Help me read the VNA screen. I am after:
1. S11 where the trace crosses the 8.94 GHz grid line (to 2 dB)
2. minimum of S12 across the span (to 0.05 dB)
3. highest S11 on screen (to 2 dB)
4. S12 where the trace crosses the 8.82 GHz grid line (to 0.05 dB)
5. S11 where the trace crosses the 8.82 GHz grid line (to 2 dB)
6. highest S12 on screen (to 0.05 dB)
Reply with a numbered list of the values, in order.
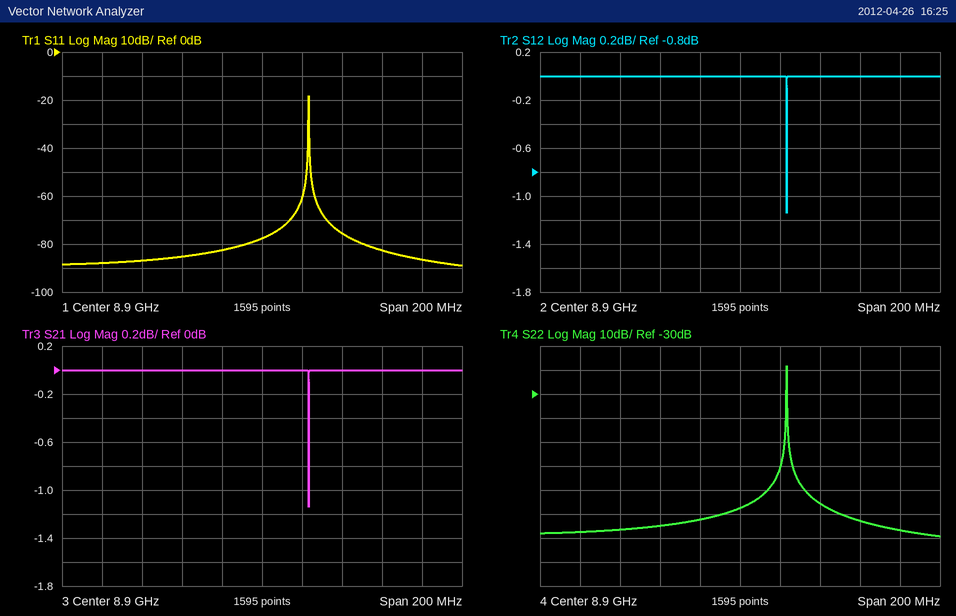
1. -76 dB
2. -1.15 dB
3. -18 dB
4. 0.00 dB
5. -88 dB
6. 0.00 dB
